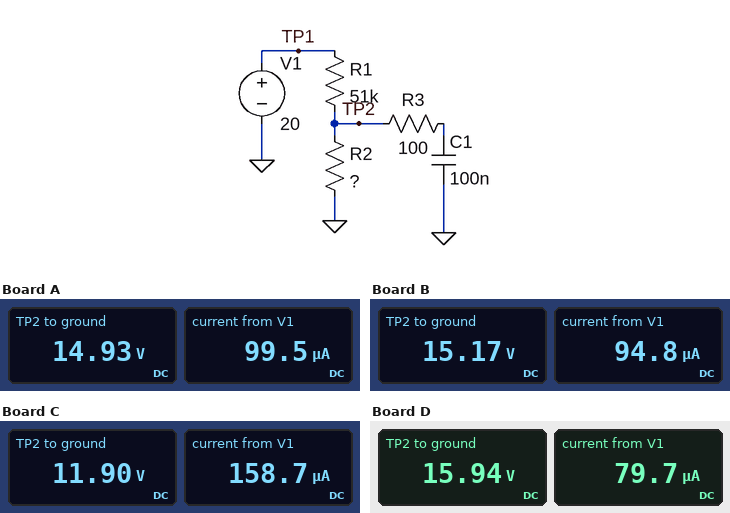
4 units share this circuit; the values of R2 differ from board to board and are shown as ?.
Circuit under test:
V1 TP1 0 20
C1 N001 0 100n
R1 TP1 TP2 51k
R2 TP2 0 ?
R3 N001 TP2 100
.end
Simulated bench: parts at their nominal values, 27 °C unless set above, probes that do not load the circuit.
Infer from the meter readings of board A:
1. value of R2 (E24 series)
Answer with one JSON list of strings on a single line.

["150 kΩ"]
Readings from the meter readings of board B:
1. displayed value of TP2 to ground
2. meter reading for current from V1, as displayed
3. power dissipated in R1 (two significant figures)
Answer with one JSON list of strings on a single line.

["15.17 V", "94.8 µA", "460 µW"]
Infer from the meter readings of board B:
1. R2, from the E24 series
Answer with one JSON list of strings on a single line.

["160 kΩ"]
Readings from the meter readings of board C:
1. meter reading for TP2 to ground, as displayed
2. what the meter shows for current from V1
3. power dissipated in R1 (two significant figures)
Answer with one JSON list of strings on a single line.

["11.90 V", "158.7 µA", "1.3 mW"]
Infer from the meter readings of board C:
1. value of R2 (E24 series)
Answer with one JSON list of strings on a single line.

["75 kΩ"]
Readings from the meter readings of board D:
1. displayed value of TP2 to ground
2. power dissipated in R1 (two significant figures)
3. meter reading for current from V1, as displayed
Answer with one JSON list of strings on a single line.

["15.94 V", "320 µW", "79.7 µA"]
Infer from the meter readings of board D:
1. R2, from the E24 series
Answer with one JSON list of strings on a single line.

["200 kΩ"]
